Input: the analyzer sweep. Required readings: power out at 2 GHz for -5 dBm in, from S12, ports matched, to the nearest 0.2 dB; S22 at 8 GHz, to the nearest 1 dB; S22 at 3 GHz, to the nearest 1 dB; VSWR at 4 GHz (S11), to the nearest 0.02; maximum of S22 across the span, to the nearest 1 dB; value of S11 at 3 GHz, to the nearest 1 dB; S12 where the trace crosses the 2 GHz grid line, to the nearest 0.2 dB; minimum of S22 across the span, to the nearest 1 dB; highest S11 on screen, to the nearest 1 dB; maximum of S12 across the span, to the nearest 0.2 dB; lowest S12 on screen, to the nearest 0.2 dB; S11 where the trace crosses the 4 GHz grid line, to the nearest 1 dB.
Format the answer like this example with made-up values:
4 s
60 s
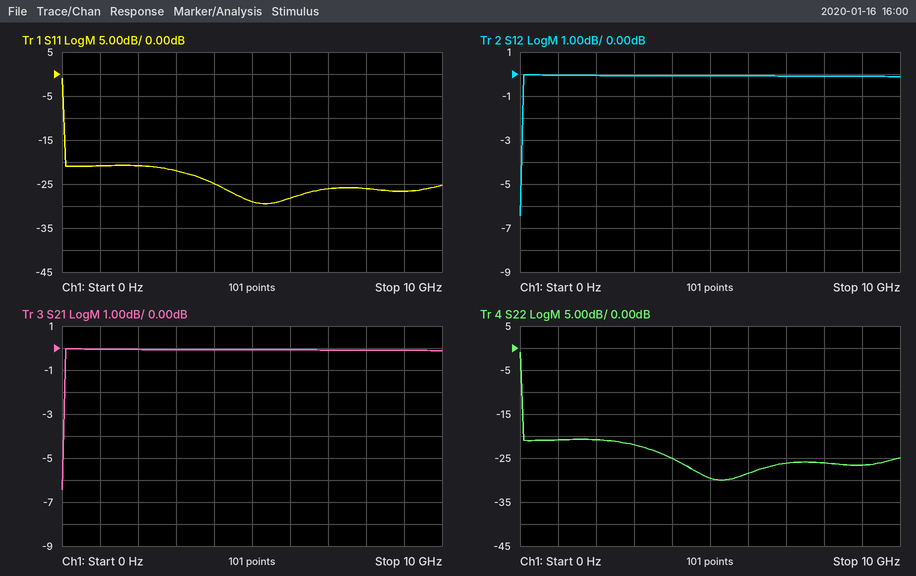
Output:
-5.0 dBm
-26 dB
-22 dB
1.12
-1 dB
-22 dB
0.0 dB
-30 dB
-1 dB
0.0 dB
-6.4 dB
-25 dB
